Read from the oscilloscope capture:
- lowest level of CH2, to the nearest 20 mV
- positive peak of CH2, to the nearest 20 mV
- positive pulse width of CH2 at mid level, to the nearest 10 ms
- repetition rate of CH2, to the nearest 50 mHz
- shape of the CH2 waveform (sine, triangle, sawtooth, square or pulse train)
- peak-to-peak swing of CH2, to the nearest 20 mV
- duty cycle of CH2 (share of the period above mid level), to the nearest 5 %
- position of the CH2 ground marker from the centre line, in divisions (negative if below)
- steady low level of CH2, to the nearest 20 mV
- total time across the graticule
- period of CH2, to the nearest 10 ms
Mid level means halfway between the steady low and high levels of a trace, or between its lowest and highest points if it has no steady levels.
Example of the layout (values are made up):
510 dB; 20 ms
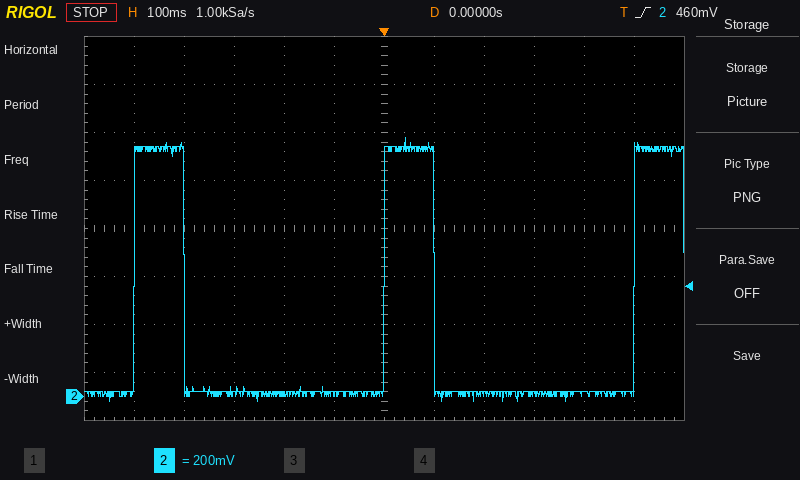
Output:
-20 mV; 1.08 V; 100 ms; 2.00 Hz; pulse train; 1.10 V; 20 %; -3.5 div; 20 mV; 1.2 s; 500 ms
